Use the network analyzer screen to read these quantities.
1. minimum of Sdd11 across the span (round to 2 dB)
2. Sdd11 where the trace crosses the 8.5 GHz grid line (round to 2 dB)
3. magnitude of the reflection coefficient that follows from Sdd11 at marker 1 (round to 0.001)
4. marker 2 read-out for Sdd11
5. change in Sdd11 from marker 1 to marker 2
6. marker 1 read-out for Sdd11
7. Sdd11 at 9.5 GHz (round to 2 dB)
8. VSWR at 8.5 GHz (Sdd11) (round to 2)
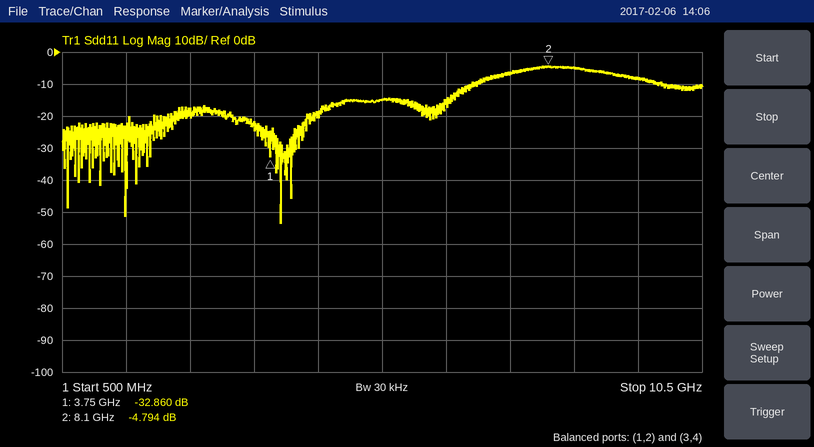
-54 dB
-4 dB
0.023
-4.794 dB
28.066 dB
-32.860 dB
-8 dB
4
